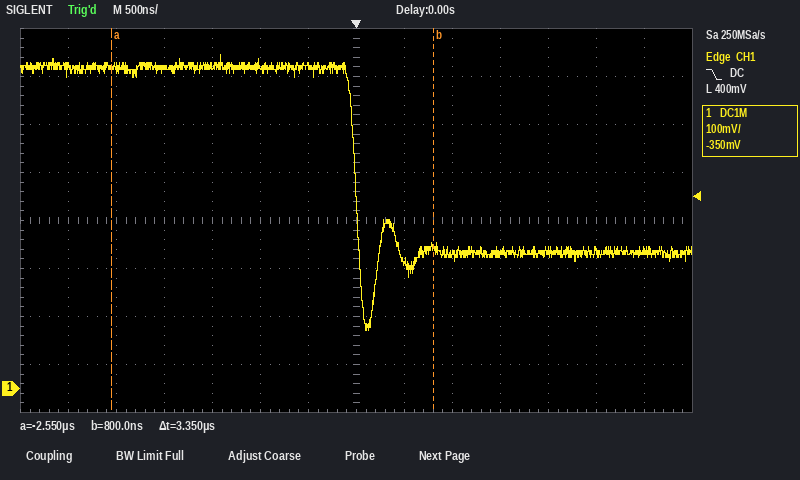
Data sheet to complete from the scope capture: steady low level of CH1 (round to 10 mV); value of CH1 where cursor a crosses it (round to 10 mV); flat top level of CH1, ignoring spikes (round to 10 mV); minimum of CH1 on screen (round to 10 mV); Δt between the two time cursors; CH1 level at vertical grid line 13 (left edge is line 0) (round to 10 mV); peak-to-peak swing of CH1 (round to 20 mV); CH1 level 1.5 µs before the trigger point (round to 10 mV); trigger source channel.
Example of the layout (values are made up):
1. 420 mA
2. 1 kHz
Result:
1. 280 mV
2. 670 mV
3. 670 mV
4. 120 mV
5. 3.35 µs
6. 290 mV
7. 580 mV
8. 670 mV
9. CH1
